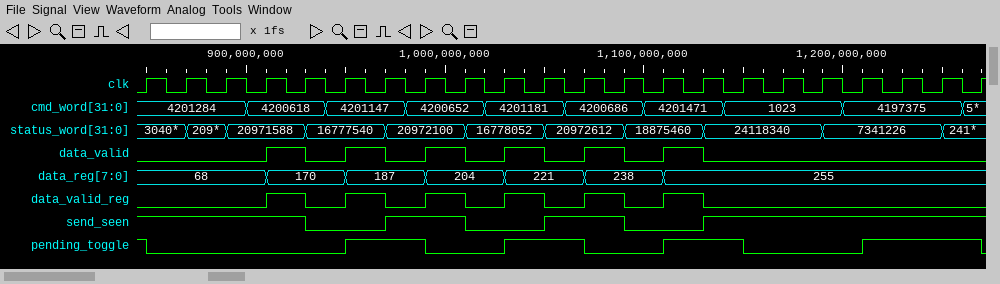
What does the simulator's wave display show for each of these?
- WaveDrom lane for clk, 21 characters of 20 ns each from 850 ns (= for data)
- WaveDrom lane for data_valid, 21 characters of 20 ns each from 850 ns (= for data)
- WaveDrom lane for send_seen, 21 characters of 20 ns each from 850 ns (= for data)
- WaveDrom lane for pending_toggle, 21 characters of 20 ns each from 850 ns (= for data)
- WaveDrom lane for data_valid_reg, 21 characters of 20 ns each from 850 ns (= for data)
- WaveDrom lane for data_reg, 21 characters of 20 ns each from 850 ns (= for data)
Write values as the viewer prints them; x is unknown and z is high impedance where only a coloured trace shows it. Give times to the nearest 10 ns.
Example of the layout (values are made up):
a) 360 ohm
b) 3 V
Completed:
a) {name: 'clk', wave: 'p....................'}
b) {name: 'data_valid', wave: '0..101010101010......'}
c) {name: 'send_seen', wave: '1...0.1.0.1.0.1......'}
d) {name: 'pending_toggle', wave: '0....1.0.1.0.1.0..1..'}
e) {name: 'data_valid_reg', wave: '0..101010101010......'}
f) {name: 'data_reg', wave: '=..=.=.=.=.=.=.......', data: '68 170 187 204 221 238 255'}
